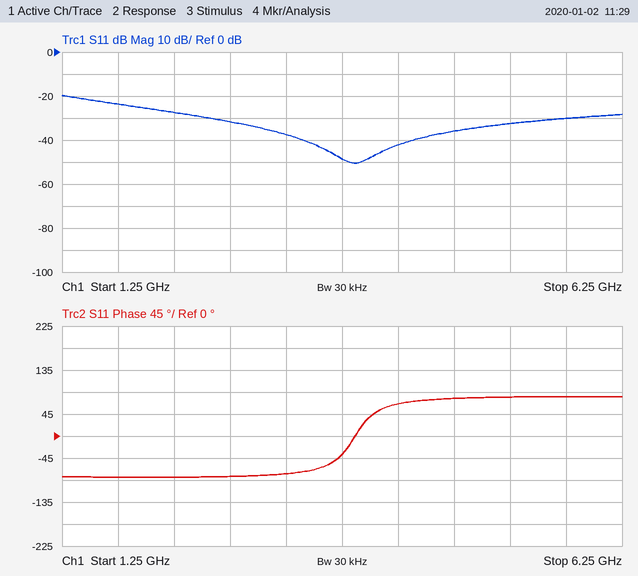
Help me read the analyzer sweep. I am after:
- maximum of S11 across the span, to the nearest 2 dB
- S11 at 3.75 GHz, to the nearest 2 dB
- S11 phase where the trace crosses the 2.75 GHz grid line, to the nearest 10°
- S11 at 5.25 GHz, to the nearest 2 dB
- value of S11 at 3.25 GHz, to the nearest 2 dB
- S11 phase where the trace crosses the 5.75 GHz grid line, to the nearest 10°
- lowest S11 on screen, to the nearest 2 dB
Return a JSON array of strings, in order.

["-20 dB", "-48 dB", "-80°", "-32 dB", "-38 dB", "80°", "-50 dB"]
